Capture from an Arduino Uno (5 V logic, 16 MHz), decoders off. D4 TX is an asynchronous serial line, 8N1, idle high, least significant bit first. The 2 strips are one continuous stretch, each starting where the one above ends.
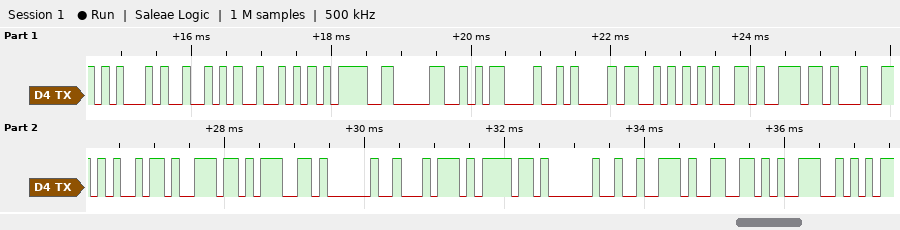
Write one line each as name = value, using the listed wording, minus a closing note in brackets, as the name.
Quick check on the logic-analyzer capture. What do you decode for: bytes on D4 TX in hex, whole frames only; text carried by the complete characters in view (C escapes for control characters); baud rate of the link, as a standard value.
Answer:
bytes on D4 TX in hex, whole frames only = 45 52 52 3D 30 0D 0A 53 65 6E 64 69 6E 67 20 74 6F 20 72 66 39
text carried by the complete characters in view = "ERR=0\r\nSending to rf9"
baud rate of the link, as a standard value = 9600 baud
